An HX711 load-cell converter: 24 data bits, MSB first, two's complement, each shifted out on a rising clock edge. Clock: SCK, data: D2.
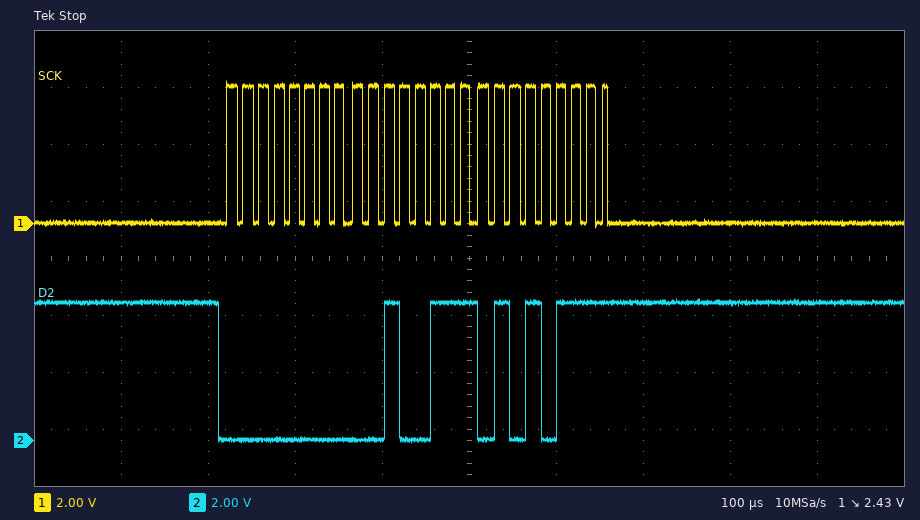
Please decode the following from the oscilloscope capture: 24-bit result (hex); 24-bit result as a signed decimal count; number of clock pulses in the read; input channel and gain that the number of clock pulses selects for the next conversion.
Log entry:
0x002757
10071
25
channel A, gain 128
